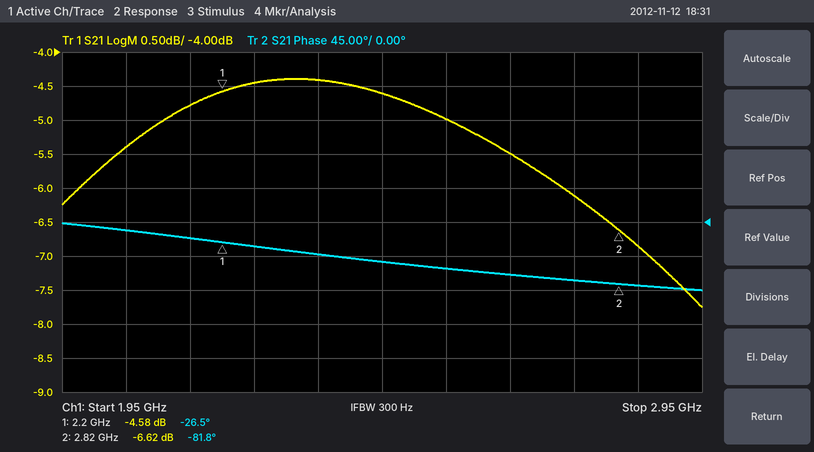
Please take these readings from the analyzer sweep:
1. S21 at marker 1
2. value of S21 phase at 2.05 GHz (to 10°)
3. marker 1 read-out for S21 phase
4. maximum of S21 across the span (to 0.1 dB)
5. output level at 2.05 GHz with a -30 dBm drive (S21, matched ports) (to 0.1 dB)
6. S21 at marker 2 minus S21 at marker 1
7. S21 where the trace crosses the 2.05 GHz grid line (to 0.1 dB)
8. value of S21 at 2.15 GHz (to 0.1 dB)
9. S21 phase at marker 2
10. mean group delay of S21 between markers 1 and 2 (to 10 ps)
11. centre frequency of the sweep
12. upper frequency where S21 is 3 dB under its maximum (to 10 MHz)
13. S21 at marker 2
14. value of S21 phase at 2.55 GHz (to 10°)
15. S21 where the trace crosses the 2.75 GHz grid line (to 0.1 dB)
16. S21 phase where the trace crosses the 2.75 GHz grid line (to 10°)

-4.58 dB
-10°
-26.5°
-4.4 dB
-35.4 dBm
-2.04 dB
-5.4 dB
-4.8 dB
-81.8°
250 ps
2.45 GHz
2.91 GHz
-6.62 dB
-60°
-6.1 dB
-80°
